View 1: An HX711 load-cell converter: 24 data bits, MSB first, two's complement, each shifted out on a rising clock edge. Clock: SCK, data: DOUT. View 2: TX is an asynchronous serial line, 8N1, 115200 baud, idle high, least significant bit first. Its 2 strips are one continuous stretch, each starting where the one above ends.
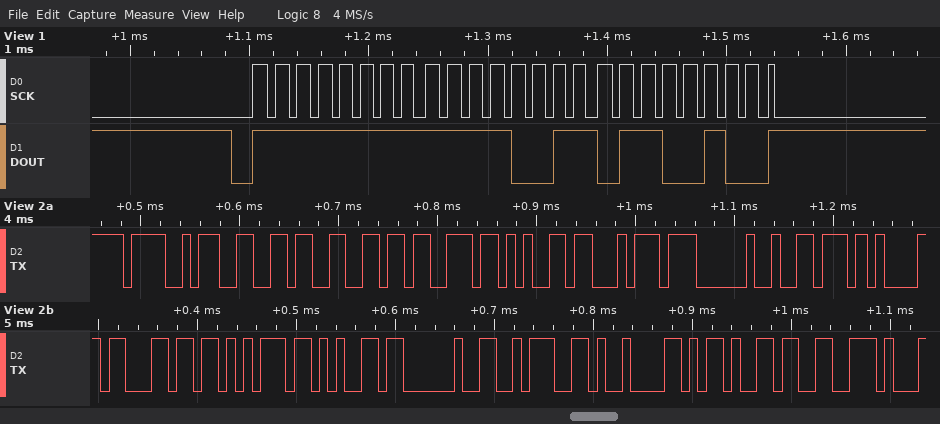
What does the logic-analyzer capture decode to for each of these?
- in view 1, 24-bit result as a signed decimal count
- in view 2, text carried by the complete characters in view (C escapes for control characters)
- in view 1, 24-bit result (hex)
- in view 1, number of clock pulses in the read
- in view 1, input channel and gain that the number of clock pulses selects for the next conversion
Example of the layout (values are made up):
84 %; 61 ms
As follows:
-3228; "Offset value :\t-3"; 0xFFF364; 25; channel A, gain 128
